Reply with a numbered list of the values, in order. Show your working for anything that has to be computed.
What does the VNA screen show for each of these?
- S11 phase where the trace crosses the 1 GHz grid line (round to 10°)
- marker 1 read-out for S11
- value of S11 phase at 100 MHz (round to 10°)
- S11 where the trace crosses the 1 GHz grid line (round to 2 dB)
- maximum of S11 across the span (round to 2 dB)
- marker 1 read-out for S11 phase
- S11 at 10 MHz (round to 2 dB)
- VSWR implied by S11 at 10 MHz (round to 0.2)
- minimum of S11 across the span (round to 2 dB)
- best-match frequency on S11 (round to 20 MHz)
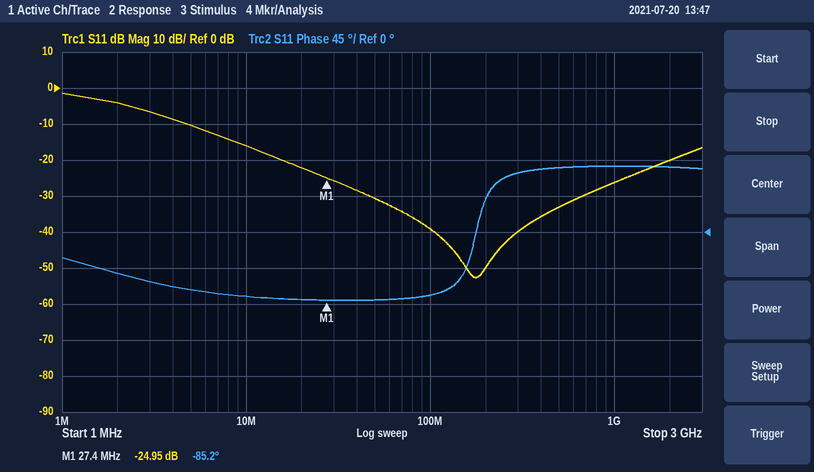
1. 80°
2. -24.95 dB
3. -80°
4. -26 dB
5. -2 dB
6. -85.2°
7. -16 dB
8. |Γ| = 10^(-16/20) = 0.1585; VSWR = (1 + 0.1585)/(1 − 0.1585) ≈ 1.4
9. -52 dB
10. 180 MHz
